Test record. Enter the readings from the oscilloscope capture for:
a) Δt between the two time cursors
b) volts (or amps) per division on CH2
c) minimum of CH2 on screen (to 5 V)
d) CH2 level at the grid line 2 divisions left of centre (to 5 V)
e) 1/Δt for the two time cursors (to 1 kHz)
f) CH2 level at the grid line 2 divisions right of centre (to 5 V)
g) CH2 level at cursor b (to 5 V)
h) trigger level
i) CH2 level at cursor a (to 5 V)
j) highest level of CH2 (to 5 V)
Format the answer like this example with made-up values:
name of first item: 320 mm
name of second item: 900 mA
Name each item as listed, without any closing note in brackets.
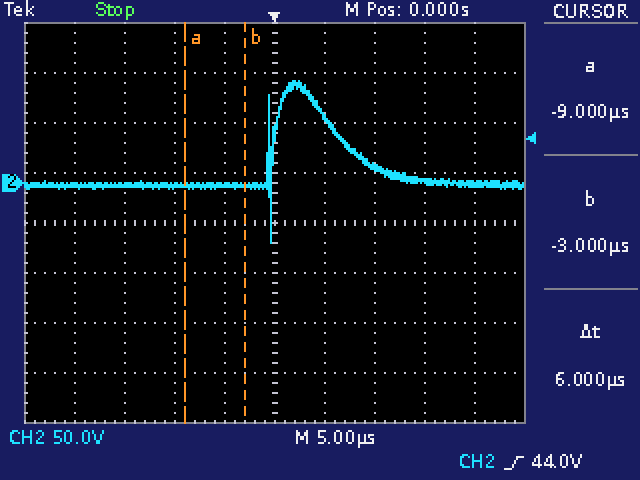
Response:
Δt between the two time cursors: 6 µs
volts (or amps) per division on CH2: 50 V
minimum of CH2 on screen: -60 V
CH2 level at the grid line 2 divisions left of centre: -5 V
1/Δt for the two time cursors: 167 kHz
CH2 level at the grid line 2 divisions right of centre: 15 V
CH2 level at cursor b: -5 V
trigger level: 44.0 V
CH2 level at cursor a: -5 V
highest level of CH2: 100 V
